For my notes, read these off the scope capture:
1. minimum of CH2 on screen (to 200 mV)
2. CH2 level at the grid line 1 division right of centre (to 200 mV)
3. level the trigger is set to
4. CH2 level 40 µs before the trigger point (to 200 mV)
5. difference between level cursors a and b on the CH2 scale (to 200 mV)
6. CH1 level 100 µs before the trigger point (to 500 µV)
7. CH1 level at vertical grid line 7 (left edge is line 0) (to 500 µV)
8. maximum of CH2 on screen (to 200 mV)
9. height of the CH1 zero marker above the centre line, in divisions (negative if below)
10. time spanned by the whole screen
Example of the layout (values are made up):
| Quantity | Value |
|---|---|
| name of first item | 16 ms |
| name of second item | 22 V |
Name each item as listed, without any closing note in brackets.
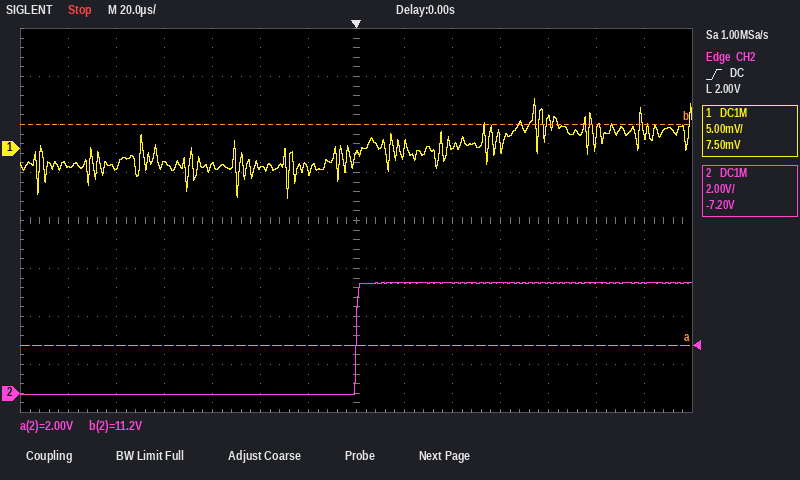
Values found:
| Quantity | Value |
|---|---|
| minimum of CH2 on screen | 0.0 V |
| CH2 level at the grid line 1 division right of centre | 4.6 V |
| level the trigger is set to | 2.00 V |
| CH2 level 40 µs before the trigger point | 0.0 V |
| difference between level cursors a and b on the CH2 scale | 9.2 V |
| CH1 level 100 µs before the trigger point | -2.0 mV |
| CH1 level at vertical grid line 7 (left edge is line 0) | -500 µV |
| maximum of CH2 on screen | 4.6 V |
| height of the CH1 zero marker above the centre line, in divisions | +1.5 div |
| time spanned by the whole screen | 280 µs |
